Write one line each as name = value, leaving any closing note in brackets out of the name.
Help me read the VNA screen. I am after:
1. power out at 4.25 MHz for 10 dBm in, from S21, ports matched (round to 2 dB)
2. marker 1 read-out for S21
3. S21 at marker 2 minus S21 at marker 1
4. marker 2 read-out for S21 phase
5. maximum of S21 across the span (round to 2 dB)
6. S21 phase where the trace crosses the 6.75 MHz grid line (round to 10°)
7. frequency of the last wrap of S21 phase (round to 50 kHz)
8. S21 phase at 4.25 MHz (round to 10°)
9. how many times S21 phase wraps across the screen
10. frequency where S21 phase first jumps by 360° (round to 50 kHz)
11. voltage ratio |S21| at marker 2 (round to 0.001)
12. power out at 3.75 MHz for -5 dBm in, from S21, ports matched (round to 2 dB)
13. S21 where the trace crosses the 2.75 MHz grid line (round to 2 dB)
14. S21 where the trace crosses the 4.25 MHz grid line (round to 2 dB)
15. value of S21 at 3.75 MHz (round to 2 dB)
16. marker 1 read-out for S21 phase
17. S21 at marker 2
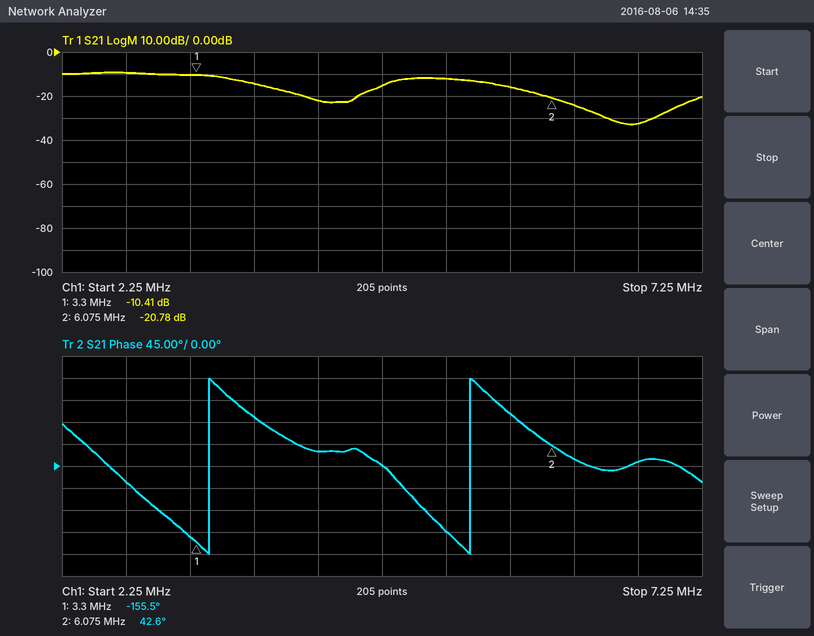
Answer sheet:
power out at 4.25 MHz for 10 dBm in, from S21, ports matched = -12 dBm
marker 1 read-out for S21 = -10.41 dB
S21 at marker 2 minus S21 at marker 1 = -10.37 dB
marker 2 read-out for S21 phase = 42.6°
maximum of S21 across the span = -10 dB
S21 phase where the trace crosses the 6.75 MHz grid line = 10°
frequency of the last wrap of S21 phase = 5.45 MHz
S21 phase at 4.25 MHz = 30°
how many times S21 phase wraps across the screen = 2
frequency where S21 phase first jumps by 360° = 3.40 MHz
voltage ratio |S21| at marker 2 = 0.091
power out at 3.75 MHz for -5 dBm in, from S21, ports matched = -20 dBm
S21 where the trace crosses the 2.75 MHz grid line = -10 dB
S21 where the trace crosses the 4.25 MHz grid line = -22 dB
value of S21 at 3.75 MHz = -14 dB
marker 1 read-out for S21 phase = -155.5°
S21 at marker 2 = -20.78 dB
